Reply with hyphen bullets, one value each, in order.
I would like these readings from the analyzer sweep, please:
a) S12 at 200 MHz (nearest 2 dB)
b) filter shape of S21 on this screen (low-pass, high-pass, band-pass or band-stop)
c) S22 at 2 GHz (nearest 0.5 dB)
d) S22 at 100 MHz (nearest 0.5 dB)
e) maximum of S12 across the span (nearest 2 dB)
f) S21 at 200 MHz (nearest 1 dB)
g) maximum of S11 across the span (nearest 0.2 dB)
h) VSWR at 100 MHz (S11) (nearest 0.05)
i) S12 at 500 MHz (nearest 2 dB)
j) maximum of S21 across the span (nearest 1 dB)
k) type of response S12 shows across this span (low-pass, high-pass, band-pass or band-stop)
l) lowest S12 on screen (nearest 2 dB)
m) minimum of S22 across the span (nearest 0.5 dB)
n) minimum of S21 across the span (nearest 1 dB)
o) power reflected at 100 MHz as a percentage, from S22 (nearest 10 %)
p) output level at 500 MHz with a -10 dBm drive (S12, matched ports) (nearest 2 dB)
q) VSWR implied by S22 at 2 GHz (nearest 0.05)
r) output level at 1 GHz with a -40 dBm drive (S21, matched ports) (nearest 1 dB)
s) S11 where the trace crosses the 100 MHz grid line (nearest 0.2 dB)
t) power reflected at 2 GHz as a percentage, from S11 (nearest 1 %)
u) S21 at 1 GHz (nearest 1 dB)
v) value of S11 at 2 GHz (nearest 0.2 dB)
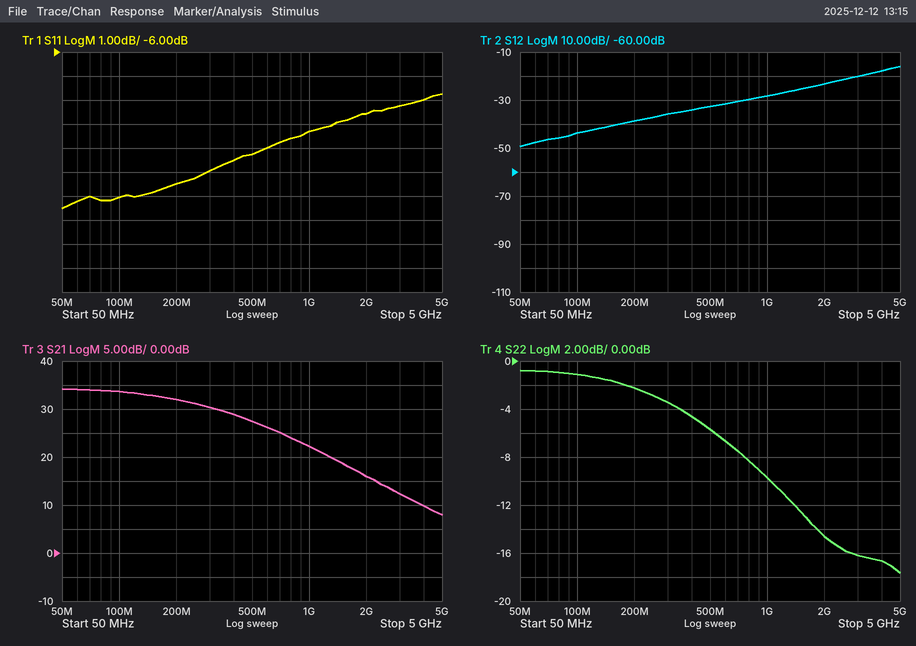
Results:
- -38 dB
- low-pass
- -14.5 dB
- -1.0 dB
- -16 dB
- 32 dB
- -7.8 dB
- 1.65
- -32 dB
- 34 dB
- high-pass
- -50 dB
- -17.5 dB
- 8 dB
- 80 %
- -42 dBm
- 1.45
- -18 dBm
- -12.0 dB
- 14 %
- 22 dB
- -8.6 dB
